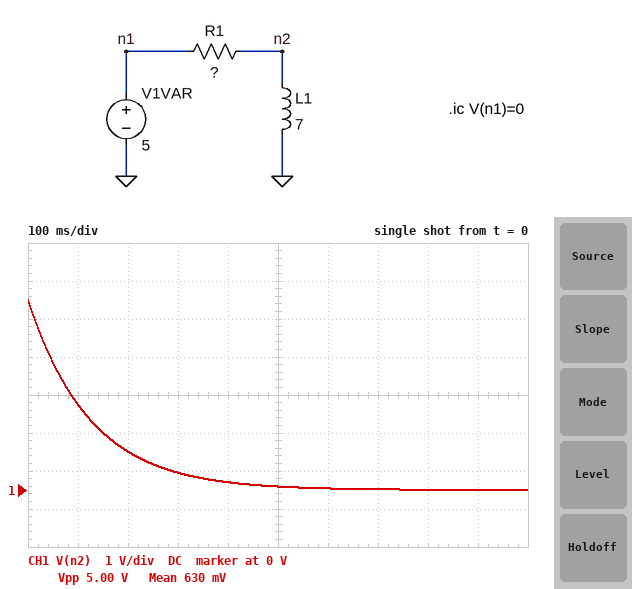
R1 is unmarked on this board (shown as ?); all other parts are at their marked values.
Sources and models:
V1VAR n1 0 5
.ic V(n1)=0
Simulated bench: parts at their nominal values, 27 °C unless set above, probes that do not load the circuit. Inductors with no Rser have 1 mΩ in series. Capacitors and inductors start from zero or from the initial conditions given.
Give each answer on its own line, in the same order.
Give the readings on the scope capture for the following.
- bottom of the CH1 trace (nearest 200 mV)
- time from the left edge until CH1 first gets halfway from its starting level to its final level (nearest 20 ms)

0 V
80 ms
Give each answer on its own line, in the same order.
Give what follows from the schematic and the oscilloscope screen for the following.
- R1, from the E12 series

56 Ω
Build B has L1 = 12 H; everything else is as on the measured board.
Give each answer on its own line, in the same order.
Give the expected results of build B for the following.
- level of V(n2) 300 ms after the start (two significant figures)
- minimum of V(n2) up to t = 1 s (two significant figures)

1.2 V
47 mV
